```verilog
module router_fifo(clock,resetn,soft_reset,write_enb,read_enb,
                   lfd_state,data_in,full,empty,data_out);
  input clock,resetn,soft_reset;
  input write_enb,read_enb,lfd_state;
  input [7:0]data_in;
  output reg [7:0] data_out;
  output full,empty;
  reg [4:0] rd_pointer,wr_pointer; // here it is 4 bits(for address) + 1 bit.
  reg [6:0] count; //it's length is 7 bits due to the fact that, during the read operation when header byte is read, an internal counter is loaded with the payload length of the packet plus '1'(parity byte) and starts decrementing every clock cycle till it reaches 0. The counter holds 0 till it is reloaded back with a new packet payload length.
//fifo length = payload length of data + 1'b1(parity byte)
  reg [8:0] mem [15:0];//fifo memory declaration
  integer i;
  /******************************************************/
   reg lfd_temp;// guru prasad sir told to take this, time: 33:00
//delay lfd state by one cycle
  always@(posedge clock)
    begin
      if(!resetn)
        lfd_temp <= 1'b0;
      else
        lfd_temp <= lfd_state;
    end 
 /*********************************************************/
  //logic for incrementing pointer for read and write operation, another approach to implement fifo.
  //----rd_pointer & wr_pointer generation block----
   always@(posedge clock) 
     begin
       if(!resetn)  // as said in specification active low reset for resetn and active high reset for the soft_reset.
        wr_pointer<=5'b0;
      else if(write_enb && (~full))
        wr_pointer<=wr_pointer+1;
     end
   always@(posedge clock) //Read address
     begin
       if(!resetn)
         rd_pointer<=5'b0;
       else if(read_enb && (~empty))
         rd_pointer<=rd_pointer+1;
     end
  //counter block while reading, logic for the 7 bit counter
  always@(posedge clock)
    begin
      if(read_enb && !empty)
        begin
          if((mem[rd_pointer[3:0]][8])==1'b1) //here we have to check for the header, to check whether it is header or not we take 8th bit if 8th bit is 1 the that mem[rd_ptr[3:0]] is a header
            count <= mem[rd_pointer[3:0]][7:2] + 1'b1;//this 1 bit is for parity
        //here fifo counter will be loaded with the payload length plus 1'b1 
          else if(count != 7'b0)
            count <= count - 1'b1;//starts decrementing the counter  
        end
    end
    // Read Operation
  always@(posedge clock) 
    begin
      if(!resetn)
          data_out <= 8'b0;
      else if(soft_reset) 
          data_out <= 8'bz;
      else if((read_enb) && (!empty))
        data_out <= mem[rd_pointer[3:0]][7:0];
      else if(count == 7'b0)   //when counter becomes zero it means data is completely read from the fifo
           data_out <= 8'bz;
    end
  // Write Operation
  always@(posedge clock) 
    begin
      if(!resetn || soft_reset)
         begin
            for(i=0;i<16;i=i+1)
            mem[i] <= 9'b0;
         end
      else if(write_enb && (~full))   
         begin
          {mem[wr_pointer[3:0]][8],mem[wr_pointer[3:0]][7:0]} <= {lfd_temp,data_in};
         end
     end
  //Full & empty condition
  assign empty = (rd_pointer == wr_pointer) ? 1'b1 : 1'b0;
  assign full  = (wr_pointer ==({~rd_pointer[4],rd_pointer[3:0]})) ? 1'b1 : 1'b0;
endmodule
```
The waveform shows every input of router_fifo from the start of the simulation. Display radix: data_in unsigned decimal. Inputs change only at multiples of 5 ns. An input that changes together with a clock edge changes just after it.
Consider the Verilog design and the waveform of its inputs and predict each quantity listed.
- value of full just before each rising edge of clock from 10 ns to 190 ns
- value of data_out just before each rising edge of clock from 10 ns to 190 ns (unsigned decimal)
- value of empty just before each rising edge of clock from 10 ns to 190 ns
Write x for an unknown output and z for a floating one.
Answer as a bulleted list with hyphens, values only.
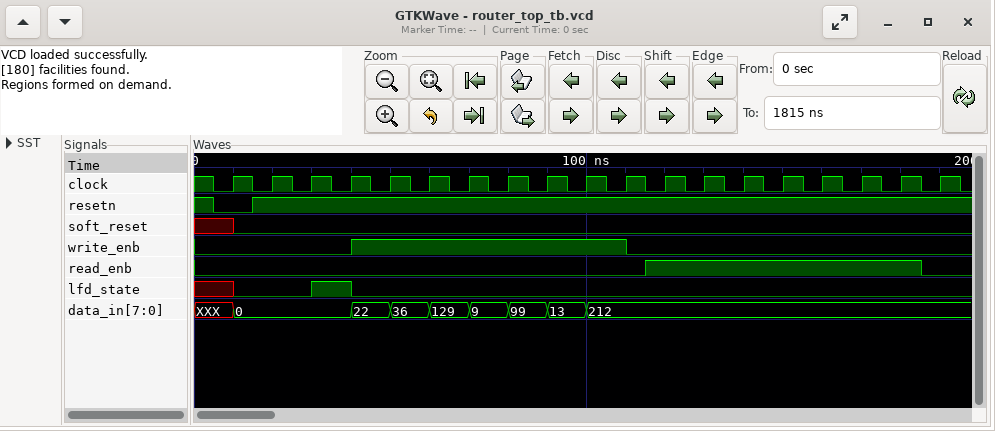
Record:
- x 0 0 0 0 0 0 0 0 0 0 0 0 0 0 0 0 0 0
- x, 0, 0, 0, 0, 0, 0, 0, 0, 0, 0, 0, 22, 36, 129, 9, 99, 13, 212
- x 1 1 1 1 0 0 0 0 0 0 0 0 0 0 0 0 0 1
